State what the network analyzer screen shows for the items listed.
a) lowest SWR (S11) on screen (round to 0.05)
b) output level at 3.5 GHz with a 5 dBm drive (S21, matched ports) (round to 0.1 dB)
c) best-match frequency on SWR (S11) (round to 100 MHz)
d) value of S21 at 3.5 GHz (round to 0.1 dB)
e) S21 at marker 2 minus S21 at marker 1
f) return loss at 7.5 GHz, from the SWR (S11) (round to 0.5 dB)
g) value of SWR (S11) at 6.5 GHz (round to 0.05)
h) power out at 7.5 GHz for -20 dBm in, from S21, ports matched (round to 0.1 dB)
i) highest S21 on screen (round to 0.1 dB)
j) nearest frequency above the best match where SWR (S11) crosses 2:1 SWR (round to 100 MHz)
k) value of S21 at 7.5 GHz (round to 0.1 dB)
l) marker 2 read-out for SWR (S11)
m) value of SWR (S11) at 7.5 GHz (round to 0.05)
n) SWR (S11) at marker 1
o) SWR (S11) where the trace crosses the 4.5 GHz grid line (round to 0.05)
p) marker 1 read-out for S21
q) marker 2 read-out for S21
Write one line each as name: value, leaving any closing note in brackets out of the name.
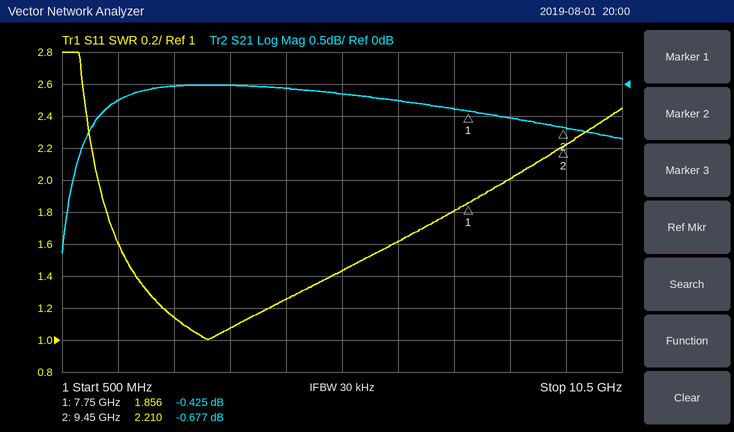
lowest SWR (S11) on screen: 1.00
output level at 3.5 GHz with a 5 dBm drive (S21, matched ports): 5.0 dBm
best-match frequency on SWR (S11): 3.1 GHz
value of S21 at 3.5 GHz: 0.0 dB
S21 at marker 2 minus S21 at marker 1: -0.252 dB
return loss at 7.5 GHz, from the SWR (S11): 11.0 dB
value of SWR (S11) at 6.5 GHz: 1.60
power out at 7.5 GHz for -20 dBm in, from S21, ports matched: -20.4 dBm
highest S21 on screen: 0.0 dB
nearest frequency above the best match where SWR (S11) crosses 2:1 SWR: 8.5 GHz
value of S21 at 7.5 GHz: -0.4 dB
marker 2 read-out for SWR: 2.210
value of SWR (S11) at 7.5 GHz: 1.80
SWR (S11) at marker 1: 1.856
SWR (S11) where the trace crosses the 4.5 GHz grid line: 1.25
marker 1 read-out for S21: -0.425 dB
marker 2 read-out for S21: -0.677 dB
